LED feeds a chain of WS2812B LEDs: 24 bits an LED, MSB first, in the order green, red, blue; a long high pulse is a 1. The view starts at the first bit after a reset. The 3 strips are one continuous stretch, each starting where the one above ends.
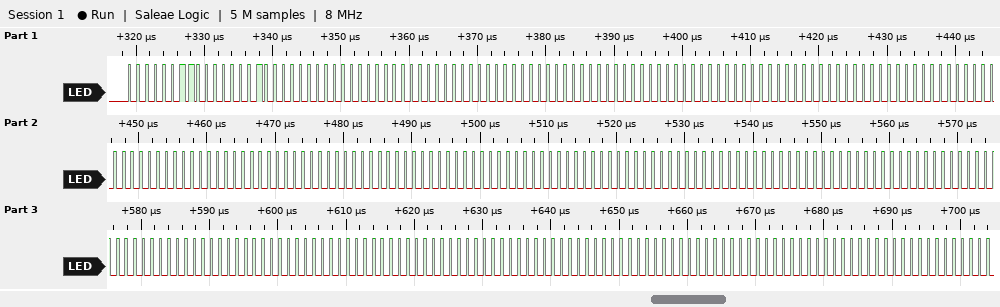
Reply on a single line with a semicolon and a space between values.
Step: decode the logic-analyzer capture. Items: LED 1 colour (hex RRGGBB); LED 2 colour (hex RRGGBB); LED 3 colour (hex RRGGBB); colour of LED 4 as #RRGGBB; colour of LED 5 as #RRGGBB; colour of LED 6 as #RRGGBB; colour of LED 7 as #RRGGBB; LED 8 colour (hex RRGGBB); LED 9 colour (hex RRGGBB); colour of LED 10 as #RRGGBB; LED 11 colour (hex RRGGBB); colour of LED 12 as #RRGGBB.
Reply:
#010300; #000000; #000000; #000000; #000000; #000000; #000000; #000000; #000000; #000000; #000000; #000000
